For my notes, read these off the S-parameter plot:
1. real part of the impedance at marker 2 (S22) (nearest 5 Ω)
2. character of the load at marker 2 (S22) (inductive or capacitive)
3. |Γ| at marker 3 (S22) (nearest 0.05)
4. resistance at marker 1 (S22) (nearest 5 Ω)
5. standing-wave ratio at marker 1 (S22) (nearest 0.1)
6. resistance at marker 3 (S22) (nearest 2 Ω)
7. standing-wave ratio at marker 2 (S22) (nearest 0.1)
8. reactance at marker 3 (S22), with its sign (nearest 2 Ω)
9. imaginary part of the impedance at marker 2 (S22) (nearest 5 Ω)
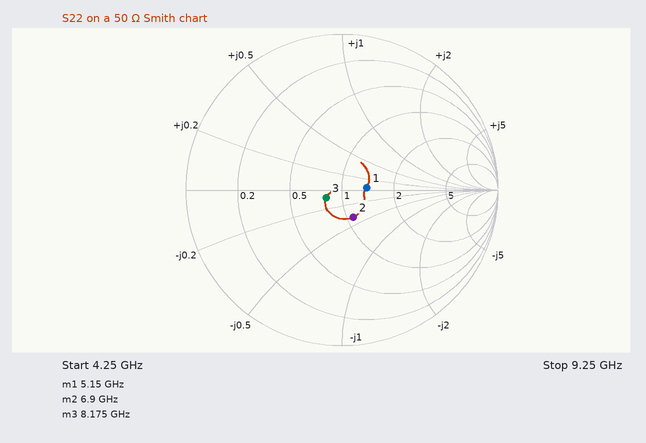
55 Ω
capacitive
0.10
70 Ω
1.4
40 Ω
1.5
-4 Ω
-20 Ω
